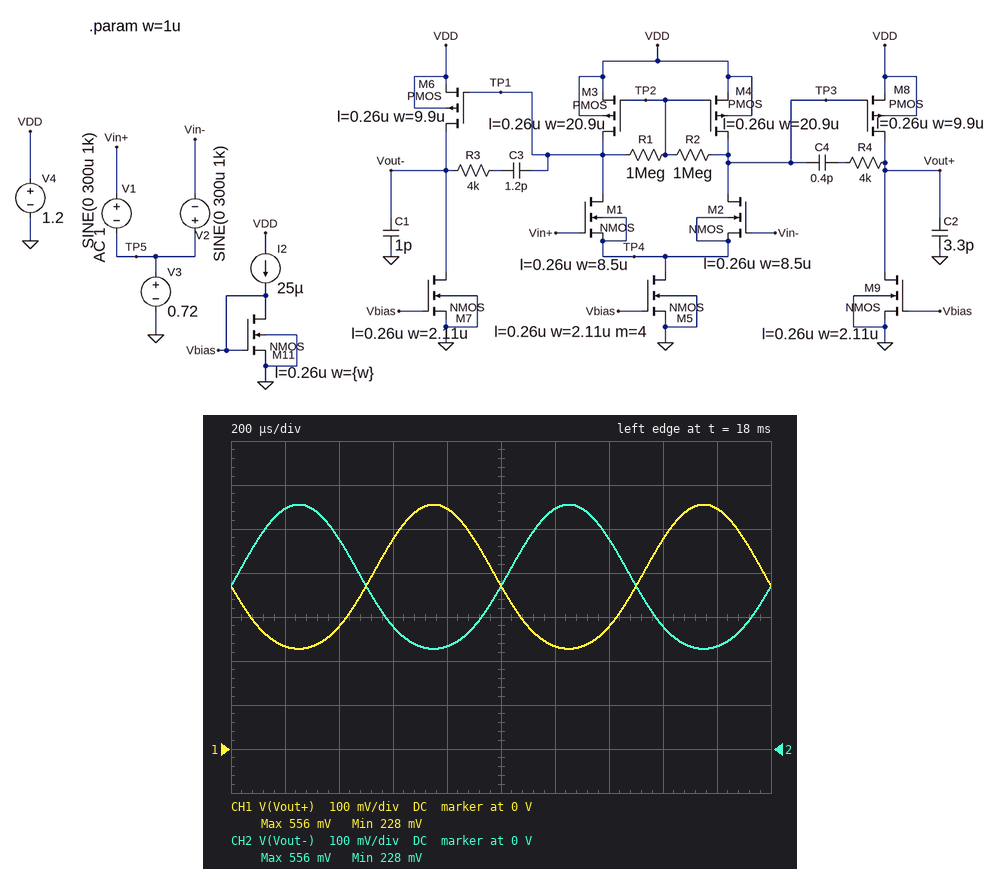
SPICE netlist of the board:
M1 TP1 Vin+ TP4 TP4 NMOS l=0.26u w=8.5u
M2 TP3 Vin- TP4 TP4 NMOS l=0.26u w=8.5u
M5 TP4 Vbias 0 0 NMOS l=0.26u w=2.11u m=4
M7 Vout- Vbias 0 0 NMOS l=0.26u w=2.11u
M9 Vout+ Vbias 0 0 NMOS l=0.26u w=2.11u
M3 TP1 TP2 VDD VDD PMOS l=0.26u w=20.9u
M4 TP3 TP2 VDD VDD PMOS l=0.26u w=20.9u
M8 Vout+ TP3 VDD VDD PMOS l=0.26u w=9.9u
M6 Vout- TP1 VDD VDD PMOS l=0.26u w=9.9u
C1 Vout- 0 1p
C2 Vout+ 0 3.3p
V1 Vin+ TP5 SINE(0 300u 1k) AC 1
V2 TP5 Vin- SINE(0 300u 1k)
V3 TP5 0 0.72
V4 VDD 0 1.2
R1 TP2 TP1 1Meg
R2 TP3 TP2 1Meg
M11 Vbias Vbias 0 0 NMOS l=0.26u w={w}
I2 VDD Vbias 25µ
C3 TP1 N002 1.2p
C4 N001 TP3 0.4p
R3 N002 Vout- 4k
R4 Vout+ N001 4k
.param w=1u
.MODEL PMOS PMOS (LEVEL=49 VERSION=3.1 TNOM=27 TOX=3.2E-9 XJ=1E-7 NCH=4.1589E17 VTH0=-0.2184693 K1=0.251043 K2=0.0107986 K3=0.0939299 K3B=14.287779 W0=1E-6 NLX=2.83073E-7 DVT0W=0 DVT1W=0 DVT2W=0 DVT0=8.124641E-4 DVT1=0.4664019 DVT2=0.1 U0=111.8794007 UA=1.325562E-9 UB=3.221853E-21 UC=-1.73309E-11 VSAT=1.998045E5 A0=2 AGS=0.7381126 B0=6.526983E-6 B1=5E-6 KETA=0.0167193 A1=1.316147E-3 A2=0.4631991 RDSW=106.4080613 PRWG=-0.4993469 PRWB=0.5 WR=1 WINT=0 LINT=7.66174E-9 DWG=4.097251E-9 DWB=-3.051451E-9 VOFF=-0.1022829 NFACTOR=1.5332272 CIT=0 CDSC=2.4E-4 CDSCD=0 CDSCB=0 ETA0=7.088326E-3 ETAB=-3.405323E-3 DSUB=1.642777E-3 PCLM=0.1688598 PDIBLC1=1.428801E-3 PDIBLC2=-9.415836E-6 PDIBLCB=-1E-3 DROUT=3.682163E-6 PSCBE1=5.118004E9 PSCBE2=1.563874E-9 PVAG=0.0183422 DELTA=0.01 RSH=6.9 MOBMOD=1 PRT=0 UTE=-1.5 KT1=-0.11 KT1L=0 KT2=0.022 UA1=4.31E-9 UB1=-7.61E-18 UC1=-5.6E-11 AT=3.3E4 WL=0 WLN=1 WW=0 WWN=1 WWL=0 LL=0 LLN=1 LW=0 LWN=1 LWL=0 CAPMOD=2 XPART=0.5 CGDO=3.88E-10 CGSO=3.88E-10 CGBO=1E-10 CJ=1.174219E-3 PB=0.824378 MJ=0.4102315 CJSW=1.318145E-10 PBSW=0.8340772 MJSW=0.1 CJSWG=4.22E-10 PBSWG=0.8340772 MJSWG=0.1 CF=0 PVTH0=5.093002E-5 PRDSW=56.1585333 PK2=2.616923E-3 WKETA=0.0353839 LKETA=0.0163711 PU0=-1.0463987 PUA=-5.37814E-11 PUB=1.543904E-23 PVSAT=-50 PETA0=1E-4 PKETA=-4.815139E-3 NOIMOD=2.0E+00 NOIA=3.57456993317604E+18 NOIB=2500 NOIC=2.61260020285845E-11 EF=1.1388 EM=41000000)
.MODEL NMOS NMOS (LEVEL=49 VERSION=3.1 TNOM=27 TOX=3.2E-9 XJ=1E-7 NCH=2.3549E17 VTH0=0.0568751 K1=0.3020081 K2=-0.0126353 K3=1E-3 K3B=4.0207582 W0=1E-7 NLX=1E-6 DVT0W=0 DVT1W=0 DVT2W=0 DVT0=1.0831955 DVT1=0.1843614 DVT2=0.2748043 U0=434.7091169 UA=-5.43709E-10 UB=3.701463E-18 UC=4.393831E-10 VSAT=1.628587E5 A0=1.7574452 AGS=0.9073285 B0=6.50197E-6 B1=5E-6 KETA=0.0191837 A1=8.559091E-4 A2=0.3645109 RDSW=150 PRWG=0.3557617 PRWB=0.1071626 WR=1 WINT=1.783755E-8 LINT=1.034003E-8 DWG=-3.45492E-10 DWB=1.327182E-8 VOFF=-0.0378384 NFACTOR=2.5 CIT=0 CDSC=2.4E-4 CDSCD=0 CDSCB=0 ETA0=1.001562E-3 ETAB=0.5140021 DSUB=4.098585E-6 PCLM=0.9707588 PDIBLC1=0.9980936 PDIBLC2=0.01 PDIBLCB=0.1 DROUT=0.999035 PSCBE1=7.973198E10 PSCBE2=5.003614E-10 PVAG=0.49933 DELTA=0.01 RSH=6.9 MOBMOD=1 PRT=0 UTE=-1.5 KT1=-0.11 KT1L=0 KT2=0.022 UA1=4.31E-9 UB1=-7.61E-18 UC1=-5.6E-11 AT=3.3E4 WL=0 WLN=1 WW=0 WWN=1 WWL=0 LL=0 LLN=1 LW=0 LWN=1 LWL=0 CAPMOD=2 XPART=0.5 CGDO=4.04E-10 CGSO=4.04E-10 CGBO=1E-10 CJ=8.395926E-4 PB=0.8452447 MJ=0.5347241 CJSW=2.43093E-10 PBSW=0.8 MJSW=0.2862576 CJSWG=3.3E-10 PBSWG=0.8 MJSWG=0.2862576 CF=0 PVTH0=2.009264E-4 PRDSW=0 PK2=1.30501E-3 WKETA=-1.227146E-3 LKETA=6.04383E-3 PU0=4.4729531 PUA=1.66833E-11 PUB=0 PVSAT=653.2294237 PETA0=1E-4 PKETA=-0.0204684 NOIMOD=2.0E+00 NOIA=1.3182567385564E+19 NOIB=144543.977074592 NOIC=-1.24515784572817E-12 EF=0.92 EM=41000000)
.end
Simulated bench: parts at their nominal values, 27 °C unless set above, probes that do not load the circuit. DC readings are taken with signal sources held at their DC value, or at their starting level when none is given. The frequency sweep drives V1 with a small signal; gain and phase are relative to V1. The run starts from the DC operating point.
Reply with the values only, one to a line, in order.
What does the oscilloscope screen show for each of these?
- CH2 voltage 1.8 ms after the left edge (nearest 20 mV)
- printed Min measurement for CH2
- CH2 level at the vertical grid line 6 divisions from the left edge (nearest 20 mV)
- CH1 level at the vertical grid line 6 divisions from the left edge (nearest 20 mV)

240 mV
228 mV
540 mV
240 mV
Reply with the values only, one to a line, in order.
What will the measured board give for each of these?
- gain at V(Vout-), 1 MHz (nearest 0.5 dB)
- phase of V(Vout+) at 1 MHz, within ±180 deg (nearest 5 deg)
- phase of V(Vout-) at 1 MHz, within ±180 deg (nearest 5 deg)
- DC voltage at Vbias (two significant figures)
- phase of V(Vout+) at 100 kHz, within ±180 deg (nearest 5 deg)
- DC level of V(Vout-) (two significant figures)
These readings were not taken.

41.0 dB
105 deg
-65 deg
500 mV
165 deg
370 mV
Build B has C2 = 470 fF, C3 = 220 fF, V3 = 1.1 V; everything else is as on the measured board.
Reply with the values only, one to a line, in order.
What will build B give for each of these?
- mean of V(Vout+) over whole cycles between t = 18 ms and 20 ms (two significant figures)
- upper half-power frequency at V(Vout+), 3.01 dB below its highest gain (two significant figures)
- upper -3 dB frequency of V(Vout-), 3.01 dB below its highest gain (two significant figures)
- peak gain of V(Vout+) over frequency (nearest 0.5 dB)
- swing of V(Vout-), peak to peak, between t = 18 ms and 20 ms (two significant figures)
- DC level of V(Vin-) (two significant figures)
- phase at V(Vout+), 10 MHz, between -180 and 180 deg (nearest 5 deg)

530 mV
3.5 MHz
2.7 MHz
25.5 dB
23 mV
1.1 V
100 deg
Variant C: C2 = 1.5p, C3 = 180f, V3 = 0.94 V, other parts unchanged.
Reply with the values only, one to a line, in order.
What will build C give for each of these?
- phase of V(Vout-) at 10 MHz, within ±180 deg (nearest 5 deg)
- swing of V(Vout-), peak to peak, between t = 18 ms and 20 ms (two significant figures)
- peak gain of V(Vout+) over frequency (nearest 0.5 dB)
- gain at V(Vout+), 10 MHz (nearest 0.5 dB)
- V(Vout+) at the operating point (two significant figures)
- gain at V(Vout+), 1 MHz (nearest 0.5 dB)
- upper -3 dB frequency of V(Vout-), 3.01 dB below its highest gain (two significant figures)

-80 deg
250 mV
46.5 dB
26.0 dB
480 mV
44.0 dB
1.3 MHz
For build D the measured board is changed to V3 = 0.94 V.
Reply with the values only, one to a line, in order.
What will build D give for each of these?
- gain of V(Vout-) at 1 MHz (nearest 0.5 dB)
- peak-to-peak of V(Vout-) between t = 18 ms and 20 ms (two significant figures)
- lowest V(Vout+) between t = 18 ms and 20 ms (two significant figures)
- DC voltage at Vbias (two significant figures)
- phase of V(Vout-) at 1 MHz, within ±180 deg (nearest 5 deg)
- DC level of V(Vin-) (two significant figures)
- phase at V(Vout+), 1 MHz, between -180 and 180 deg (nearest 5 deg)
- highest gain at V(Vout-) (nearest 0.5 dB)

40.0 dB
250 mV
360 mV
500 mV
-60 deg
940 mV
110 deg
46.5 dB
